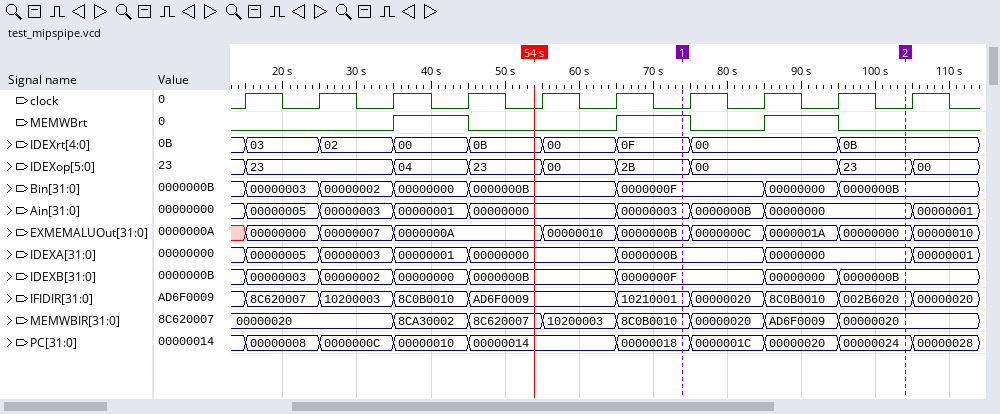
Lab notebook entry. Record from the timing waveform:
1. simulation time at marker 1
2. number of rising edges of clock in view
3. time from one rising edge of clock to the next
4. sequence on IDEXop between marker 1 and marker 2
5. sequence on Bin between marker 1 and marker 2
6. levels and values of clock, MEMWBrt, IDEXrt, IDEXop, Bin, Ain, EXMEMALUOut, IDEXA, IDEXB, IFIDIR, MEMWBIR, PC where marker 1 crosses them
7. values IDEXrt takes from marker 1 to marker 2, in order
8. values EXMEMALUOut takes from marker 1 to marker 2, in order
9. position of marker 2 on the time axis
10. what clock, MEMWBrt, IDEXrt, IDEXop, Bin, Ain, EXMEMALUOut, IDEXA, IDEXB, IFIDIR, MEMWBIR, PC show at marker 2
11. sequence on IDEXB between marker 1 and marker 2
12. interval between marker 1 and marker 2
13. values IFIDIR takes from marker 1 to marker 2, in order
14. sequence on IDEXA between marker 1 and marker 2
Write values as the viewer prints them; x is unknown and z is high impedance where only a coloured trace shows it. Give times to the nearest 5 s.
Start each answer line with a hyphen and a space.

- 75 s
- 10
- 10 s
- 2B, 00, 23
- 0000000F, 00000000, 0000000B
- clock=0, MEMWBrt=1, IDEXrt=0F, IDEXop=2B, Bin=0000000F, Ain=00000003, EXMEMALUOut=0000000B, IDEXA=0000000B, IDEXB=0000000F, IFIDIR=10210001, MEMWBIR=8C0B0010, PC=00000018
- 0F, 00, 0B
- 0000000B, 0000000C, 0000001A, 00000000
- 105 s
- clock=0, MEMWBrt=0, IDEXrt=0B, IDEXop=23, Bin=0000000B, Ain=00000000, EXMEMALUOut=00000000, IDEXA=00000000, IDEXB=0000000B, IFIDIR=002B6020, MEMWBIR=00000020, PC=00000024
- 0000000F, 00000000, 0000000B
- 30 s
- 10210001, 00000020, 8C0B0010, 002B6020
- 0000000B, 00000000
